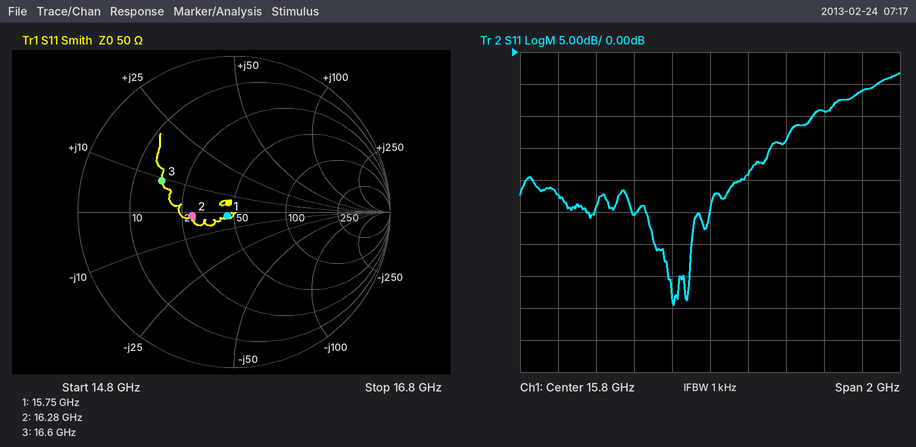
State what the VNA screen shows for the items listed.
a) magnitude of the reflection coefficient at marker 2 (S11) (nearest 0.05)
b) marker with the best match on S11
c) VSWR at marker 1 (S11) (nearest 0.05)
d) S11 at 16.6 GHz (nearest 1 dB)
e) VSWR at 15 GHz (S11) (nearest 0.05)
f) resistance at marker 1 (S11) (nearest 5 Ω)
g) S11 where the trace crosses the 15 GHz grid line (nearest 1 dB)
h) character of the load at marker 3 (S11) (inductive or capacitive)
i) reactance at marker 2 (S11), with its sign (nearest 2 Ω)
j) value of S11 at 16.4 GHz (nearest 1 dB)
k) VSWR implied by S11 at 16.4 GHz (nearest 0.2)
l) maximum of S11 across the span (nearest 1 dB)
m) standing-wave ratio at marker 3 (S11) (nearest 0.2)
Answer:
0.25
marker 1
1.10
-6 dB
1.15
45 Ω
-22 dB
inductive
-2 Ω
-9 dB
2.0
-3 dB
3.0
